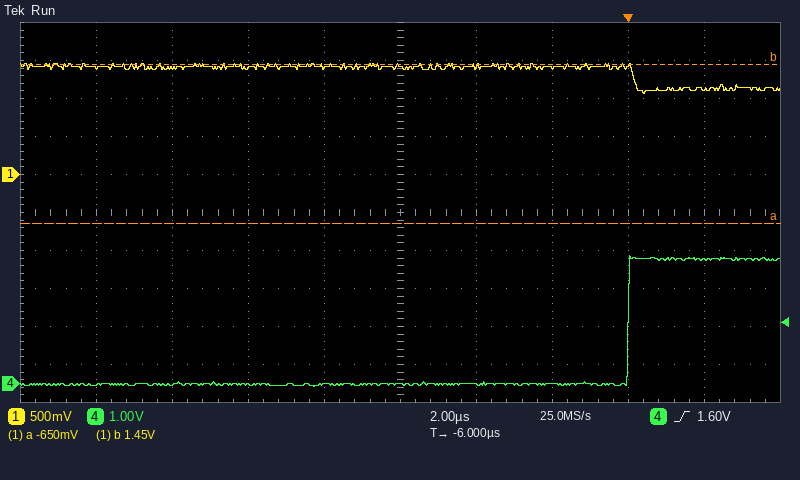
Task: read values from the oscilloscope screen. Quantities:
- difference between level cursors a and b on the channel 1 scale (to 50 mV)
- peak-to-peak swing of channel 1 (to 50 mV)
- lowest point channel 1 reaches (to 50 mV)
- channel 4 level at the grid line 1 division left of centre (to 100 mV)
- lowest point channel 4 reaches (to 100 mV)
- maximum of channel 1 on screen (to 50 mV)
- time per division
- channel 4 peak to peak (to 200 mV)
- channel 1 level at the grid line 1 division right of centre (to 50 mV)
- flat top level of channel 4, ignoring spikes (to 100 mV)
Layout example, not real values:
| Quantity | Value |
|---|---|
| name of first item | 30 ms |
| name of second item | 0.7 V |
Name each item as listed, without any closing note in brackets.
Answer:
| Quantity | Value |
|---|---|
| difference between level cursors a and b on the channel 1 scale | 2.10 V |
| peak-to-peak swing of channel 1 | 400 mV |
| lowest point channel 1 reaches | 1.05 V |
| channel 4 level at the grid line 1 division left of centre | 0.0 V |
| lowest point channel 4 reaches | -100 mV |
| maximum of channel 1 on screen | 1.45 V |
| time per division | 2 µs |
| channel 4 peak to peak | 3.4 V |
| channel 1 level at the grid line 1 division right of centre | 1.40 V |
| flat top level of channel 4, ignoring spikes | 3.3 V |
